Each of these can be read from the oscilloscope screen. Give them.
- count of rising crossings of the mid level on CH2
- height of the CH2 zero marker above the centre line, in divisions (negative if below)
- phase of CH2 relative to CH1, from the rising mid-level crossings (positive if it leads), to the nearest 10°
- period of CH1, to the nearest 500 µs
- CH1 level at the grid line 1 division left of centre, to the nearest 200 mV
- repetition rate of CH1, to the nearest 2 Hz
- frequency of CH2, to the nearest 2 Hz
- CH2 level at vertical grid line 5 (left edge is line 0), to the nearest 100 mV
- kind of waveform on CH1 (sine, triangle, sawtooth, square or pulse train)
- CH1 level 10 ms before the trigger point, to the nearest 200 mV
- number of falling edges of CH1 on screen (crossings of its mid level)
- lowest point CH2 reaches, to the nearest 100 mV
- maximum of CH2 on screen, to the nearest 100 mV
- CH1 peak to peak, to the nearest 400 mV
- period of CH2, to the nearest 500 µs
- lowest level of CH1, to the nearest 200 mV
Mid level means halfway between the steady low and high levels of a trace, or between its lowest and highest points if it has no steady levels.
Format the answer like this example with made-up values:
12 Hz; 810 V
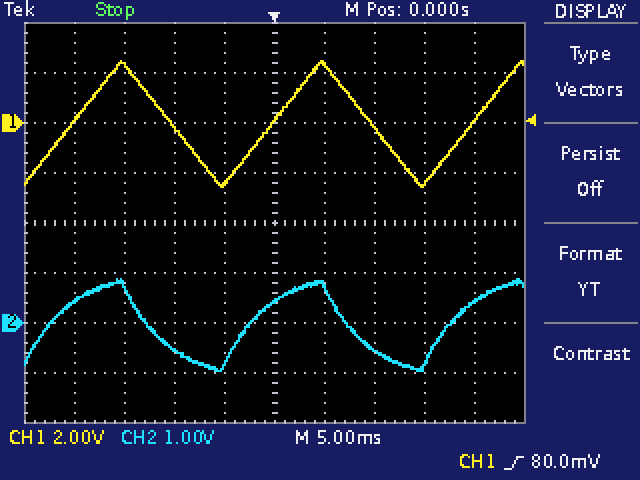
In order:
3; -2.0 div; +40°; 20.0 ms; -2.4 V; 50 Hz; 50 Hz; 400 mV; triangle; -200 mV; 2; -1.0 V; 900 mV; 5.2 V; 20.0 ms; -2.6 V
